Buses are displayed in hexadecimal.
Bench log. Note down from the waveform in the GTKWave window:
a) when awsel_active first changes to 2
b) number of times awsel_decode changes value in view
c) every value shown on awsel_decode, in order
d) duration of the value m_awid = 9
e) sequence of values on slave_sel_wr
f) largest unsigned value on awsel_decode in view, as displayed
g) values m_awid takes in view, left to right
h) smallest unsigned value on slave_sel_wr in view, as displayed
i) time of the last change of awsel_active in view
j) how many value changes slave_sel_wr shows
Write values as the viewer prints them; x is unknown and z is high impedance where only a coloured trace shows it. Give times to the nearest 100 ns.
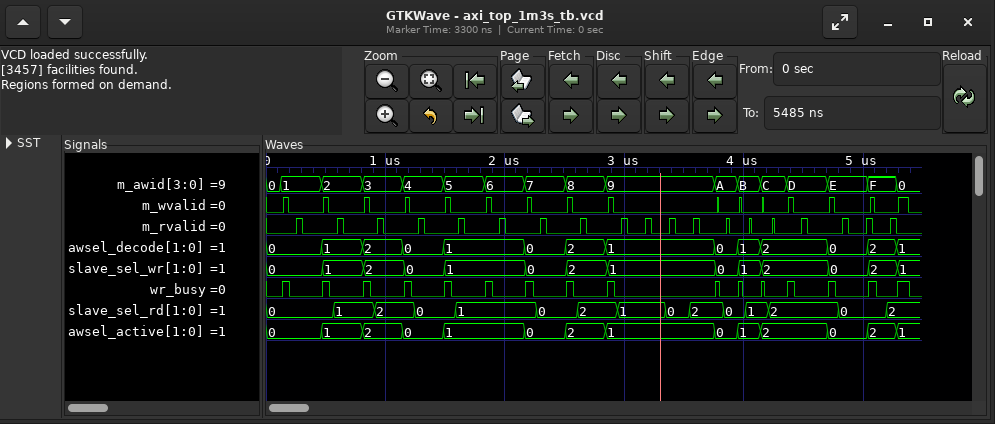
800 ns
13
0, 1, 2, 0, 1, 0, 2, 1, 0, 1, 2, 0, 2, 1
900 ns
0, 1, 2, 0, 1, 0, 2, 1, 0, 1, 2, 0, 2, 1
2
0, 1, 2, 3, 4, 5, 6, 7, 8, 9, A, B, C, D, E, F, 0
0
5300 ns
13
